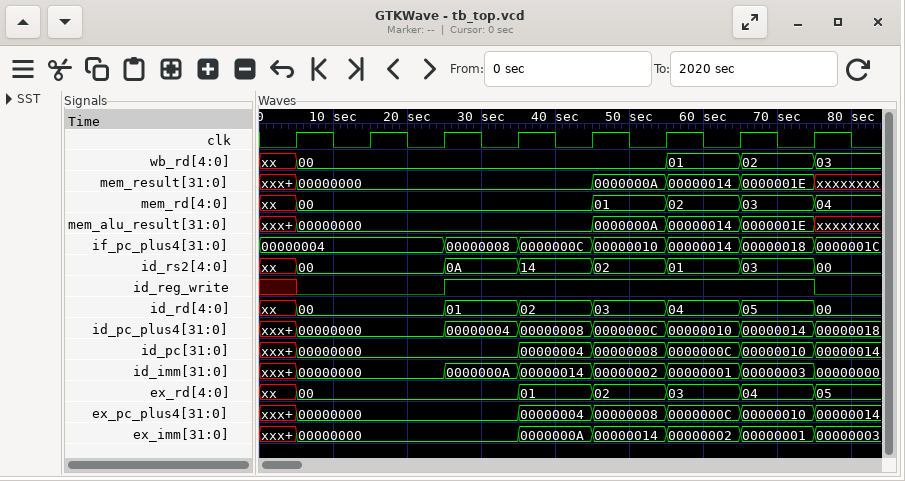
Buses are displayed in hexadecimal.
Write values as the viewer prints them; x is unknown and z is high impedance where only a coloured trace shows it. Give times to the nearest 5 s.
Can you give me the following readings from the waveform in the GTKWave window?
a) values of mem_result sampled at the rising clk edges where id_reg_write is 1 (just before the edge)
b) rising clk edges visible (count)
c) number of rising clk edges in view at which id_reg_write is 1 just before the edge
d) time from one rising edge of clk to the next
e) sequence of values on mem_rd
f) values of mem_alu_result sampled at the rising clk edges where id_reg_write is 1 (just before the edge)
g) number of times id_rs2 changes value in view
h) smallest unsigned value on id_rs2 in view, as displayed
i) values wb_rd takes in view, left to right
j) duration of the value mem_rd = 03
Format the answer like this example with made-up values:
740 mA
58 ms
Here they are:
00000000, 00000000, 0000000A, 00000014, 0000001E
8
5
10 s
xx, 00, 01, 02, 03, 04
00000000, 00000000, 0000000A, 00000014, 0000001E
7
00
xx, 00, 01, 02, 03
10 s
